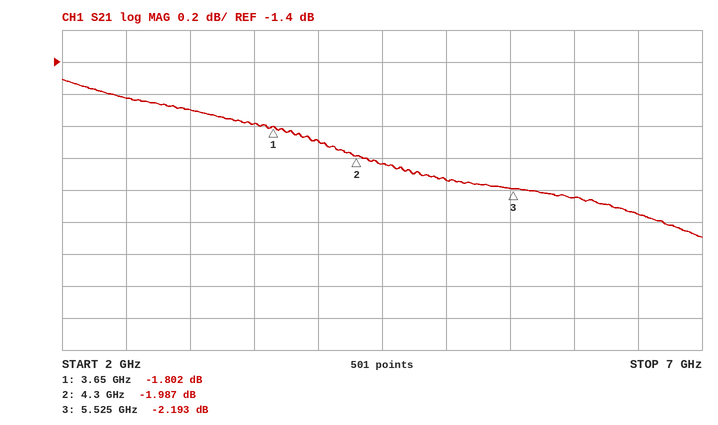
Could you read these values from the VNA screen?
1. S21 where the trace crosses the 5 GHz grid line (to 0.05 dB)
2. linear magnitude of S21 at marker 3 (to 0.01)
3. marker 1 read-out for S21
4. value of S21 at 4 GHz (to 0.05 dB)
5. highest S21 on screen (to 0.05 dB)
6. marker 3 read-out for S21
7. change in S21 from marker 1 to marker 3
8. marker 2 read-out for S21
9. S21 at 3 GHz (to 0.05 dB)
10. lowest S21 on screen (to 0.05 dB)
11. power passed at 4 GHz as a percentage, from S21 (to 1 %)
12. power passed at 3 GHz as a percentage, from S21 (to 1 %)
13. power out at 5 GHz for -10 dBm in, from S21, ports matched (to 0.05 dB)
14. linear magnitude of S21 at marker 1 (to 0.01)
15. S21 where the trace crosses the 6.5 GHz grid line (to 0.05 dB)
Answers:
-2.15 dB
0.78
-1.802 dB
-1.90 dB
-1.50 dB
-2.193 dB
-0.391 dB
-1.987 dB
-1.70 dB
-2.50 dB
65 %
68 %
-12.15 dBm
0.81
-2.35 dB
